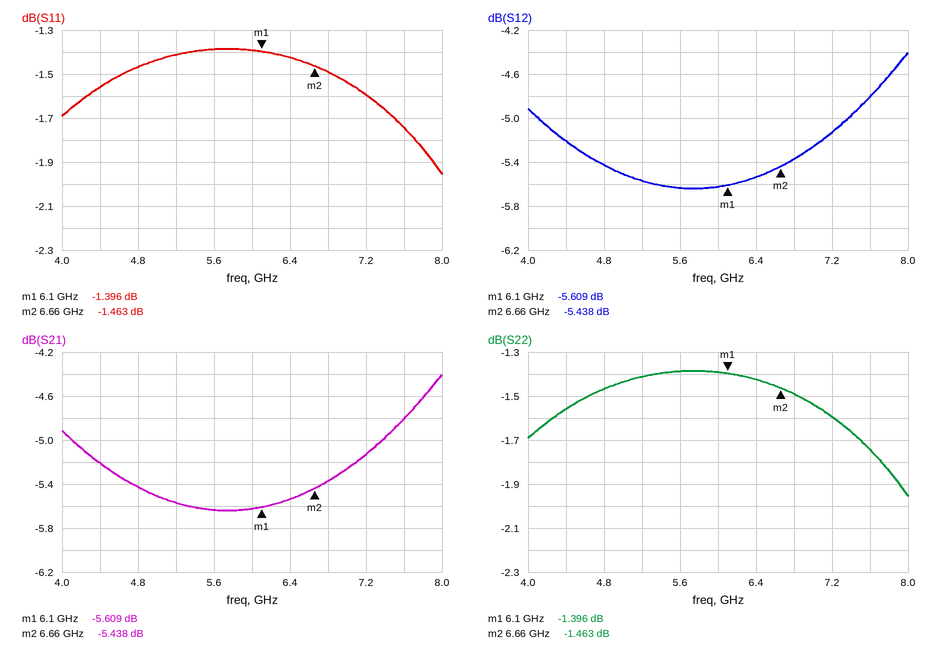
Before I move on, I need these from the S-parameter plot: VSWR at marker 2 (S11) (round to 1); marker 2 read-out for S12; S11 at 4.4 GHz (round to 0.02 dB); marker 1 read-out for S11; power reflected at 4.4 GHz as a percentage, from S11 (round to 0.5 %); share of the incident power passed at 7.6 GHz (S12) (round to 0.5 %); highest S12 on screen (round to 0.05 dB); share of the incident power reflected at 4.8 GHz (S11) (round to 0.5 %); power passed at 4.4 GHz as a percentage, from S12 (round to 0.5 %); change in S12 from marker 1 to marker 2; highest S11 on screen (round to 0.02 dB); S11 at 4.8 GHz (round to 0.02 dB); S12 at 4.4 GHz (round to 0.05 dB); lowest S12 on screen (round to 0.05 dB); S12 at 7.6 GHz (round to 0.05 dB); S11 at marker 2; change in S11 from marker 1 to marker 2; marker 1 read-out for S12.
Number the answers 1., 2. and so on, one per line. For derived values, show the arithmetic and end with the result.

1. (1 + 0.8450)/(1 − 0.8450) ≈ 12
2. -5.438 dB
3. -1.56 dB
4. -1.396 dB
5. 10^(-1.56/10) ≈ 69.8 %, so 70.0 % to the nearest 0.5 %
6. 10^(-4.8/10) ≈ 33.1 %, so 33.0 % to the nearest 0.5 %
7. -4.40 dB
8. 10^(-1.46/10) ≈ 71.4 %, so 71.5 % to the nearest 0.5 %
9. 10^(-5.2/10) ≈ 30.2 %, so 30.0 % to the nearest 0.5 %
10. -5.438 − (-5.609) = 0.171 dB
11. -1.38 dB
12. -1.46 dB
13. -5.20 dB
14. -5.65 dB
15. -4.80 dB
16. -1.463 dB
17. -1.463 − (-1.396) = -0.067 dB
18. -5.609 dB
